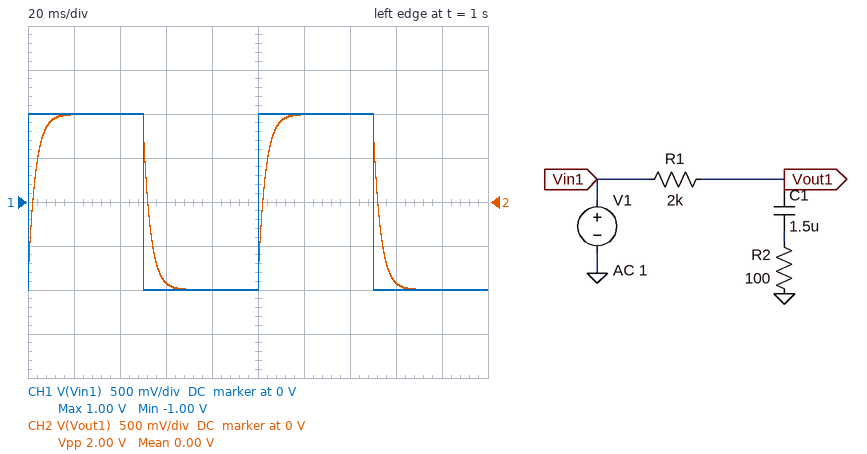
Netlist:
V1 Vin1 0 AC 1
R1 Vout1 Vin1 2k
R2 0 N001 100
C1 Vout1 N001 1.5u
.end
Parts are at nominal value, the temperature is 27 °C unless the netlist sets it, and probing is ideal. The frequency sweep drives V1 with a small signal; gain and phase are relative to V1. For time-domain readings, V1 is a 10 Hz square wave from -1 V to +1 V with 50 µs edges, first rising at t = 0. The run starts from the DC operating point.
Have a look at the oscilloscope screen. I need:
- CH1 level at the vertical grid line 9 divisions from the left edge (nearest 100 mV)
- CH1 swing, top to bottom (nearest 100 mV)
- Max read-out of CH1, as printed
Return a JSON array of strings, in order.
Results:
["-1.0 V", "2.0 V", "1.00 V"]
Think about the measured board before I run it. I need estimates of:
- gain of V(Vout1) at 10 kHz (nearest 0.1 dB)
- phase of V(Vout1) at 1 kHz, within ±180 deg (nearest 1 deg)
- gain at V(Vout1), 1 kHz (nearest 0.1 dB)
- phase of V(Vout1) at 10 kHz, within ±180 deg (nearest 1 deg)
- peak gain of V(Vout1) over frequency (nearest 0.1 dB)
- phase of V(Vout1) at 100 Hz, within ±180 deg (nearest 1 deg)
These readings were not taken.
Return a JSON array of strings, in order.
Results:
["-26.4 dB", "-44 deg", "-23.2 dB", "-6 deg", "0 dB", "-58 deg"]
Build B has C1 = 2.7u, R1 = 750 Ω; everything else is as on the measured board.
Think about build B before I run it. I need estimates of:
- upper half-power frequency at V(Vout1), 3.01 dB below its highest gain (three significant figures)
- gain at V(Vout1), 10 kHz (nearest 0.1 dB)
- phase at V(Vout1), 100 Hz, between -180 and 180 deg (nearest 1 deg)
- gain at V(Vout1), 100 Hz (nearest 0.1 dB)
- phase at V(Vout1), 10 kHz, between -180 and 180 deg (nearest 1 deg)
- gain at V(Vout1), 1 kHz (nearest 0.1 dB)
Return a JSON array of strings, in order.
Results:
["70.3 Hz", "-18.6 dB", "-46 deg", "-4.8 dB", "-3 deg", "-17.3 dB"]
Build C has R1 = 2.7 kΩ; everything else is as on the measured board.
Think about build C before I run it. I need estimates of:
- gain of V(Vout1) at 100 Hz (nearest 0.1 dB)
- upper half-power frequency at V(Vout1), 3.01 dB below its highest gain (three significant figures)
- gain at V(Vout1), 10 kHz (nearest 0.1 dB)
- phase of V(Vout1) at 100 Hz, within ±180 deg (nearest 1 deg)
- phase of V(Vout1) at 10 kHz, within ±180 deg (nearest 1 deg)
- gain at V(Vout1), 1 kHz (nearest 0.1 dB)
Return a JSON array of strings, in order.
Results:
["-9.0 dB", "37.9 Hz", "-28.9 dB", "-64 deg", "-6 deg", "-25.7 dB"]
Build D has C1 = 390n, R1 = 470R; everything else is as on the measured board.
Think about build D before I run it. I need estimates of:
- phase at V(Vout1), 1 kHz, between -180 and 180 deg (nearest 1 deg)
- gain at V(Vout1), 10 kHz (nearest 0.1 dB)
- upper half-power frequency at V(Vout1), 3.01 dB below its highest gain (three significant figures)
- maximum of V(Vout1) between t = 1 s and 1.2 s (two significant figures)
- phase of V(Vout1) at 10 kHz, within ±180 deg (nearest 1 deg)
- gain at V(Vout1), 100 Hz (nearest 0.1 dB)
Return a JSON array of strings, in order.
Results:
["-41 deg", "-14.5 dB", "739 Hz", "1.0 V", "-18 deg", "-0.1 dB"]
